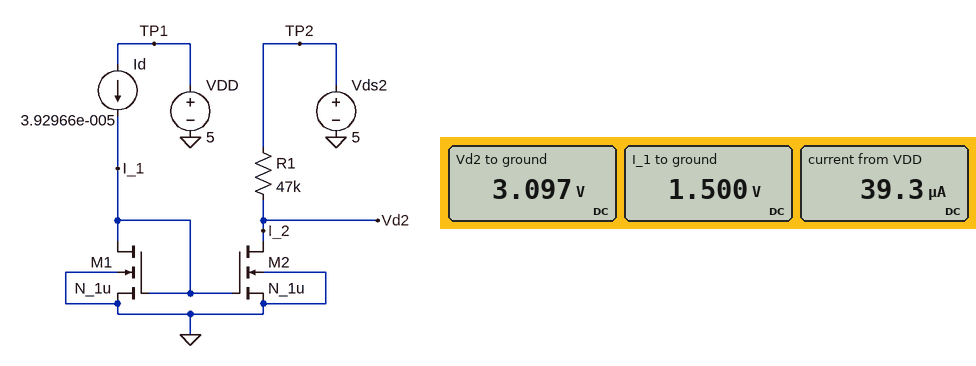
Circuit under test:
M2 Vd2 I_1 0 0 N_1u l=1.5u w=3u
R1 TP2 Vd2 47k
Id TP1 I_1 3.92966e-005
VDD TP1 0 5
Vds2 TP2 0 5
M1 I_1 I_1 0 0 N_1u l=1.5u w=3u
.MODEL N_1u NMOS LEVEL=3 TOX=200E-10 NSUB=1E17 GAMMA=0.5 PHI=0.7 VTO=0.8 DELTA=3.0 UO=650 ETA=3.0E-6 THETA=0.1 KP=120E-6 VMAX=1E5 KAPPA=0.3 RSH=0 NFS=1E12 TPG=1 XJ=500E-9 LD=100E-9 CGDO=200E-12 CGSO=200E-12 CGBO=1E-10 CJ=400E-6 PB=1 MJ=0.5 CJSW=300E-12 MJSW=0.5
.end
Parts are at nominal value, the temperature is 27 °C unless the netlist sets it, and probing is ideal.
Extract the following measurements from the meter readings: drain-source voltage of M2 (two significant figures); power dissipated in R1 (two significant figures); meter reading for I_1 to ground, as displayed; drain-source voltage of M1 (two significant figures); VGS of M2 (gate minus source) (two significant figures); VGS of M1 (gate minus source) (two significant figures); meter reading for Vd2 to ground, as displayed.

3.1 V
77 µW
1.500 V
1.5 V
1.5 V
1.5 V
3.097 V
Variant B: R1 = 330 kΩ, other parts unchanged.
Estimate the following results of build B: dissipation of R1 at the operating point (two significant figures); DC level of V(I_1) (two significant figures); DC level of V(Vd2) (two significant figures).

73 µW
1.5 V
99 mV
